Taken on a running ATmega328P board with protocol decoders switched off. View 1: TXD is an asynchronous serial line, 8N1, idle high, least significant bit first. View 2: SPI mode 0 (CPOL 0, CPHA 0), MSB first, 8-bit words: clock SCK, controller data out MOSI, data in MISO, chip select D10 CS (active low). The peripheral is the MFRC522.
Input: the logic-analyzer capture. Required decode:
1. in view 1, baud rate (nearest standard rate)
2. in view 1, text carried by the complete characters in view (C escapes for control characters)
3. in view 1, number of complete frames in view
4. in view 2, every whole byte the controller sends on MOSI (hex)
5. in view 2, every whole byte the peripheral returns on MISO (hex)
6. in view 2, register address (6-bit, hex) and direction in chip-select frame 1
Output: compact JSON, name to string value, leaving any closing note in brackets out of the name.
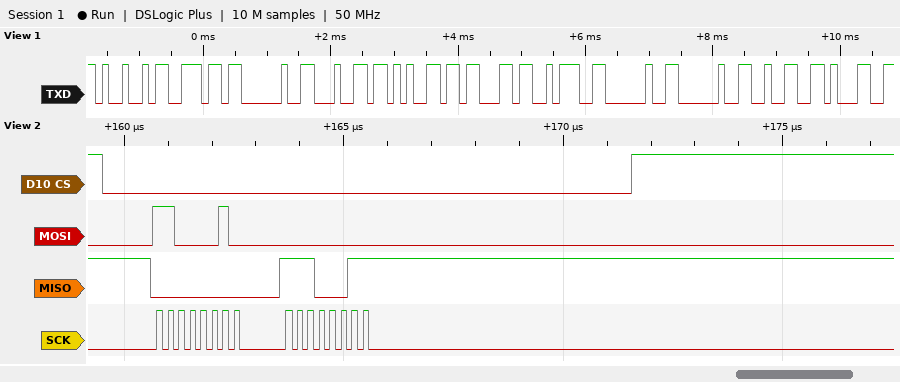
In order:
{"in view 1, baud rate": "9600 baud", "in view 1, text carried by the complete characters in view": "\"In dec:  21\"", "in view 1, number of complete frames in view": "11", "in view 2, every whole byte the controller sends on MOSI": "0xC2 0x00", "in view 2, every whole byte the peripheral returns on MISO": "0x00 0xE3", "in view 2, register address (6-bit, hex) and direction in chip-select frame 1": "0x21 read"}
